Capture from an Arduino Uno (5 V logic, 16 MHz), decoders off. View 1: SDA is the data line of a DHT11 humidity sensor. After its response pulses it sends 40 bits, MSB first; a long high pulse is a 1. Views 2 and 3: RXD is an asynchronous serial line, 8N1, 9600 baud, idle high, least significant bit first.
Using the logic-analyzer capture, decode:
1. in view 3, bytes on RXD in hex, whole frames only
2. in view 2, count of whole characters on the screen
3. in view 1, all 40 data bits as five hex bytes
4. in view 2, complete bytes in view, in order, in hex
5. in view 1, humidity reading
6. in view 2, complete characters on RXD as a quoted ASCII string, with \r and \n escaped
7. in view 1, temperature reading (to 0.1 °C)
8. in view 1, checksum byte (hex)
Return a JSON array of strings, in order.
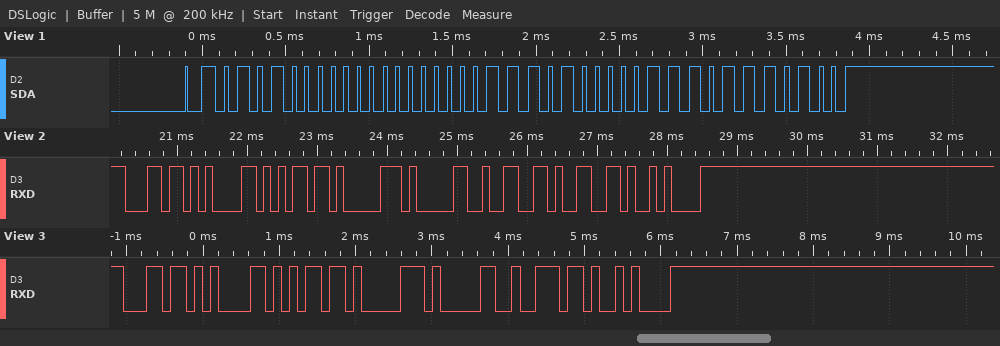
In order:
["6C 61 6D 70 30 6E 0A", "8", "50 00 1D 07 74", "6C 61 6D 70 30 66 66 0A", "80 %", "\"lamp0ff\\n\"", "29.7 °C", "0x74"]
